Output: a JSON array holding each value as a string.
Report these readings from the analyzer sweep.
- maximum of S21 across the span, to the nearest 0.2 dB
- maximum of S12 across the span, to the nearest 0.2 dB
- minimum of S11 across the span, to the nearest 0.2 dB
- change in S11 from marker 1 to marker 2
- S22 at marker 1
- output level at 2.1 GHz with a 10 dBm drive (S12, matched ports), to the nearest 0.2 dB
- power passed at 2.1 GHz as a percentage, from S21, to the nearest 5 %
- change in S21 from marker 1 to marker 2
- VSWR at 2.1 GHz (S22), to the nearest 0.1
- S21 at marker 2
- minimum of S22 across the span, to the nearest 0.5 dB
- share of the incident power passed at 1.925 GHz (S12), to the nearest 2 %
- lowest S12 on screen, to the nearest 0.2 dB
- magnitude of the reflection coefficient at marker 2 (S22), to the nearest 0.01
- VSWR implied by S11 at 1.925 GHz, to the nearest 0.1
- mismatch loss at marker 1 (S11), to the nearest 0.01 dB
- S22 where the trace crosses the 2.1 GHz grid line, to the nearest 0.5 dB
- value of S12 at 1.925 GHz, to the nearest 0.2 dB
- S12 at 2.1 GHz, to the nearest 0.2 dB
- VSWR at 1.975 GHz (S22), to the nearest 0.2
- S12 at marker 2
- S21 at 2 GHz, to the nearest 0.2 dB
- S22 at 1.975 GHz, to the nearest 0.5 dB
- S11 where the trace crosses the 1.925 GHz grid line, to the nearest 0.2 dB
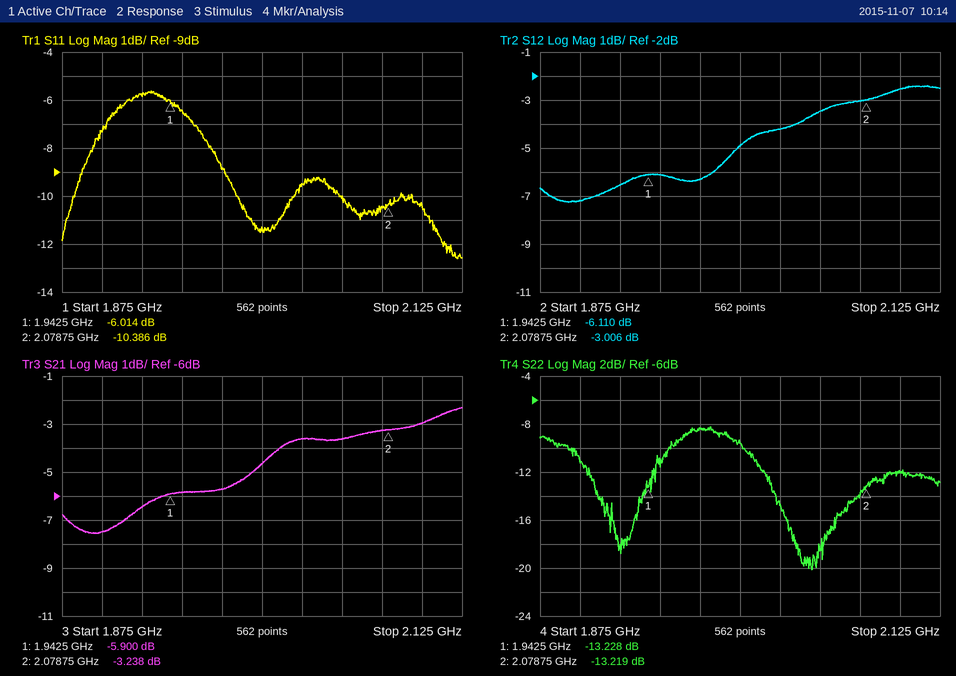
["-2.4 dB", "-2.4 dB", "-12.6 dB", "-4.372 dB", "-13.228 dB", "7.4 dBm", "50 %", "2.662 dB", "1.7", "-3.238 dB", "-20.0 dB", "22 %", "-7.2 dB", "0.22", "3.1", "1.25 dB", "-12.0 dB", "-6.6 dB", "-2.6 dB", "2.2", "-3.006 dB", "-4.6 dB", "-8.5 dB", "-5.8 dB"]
